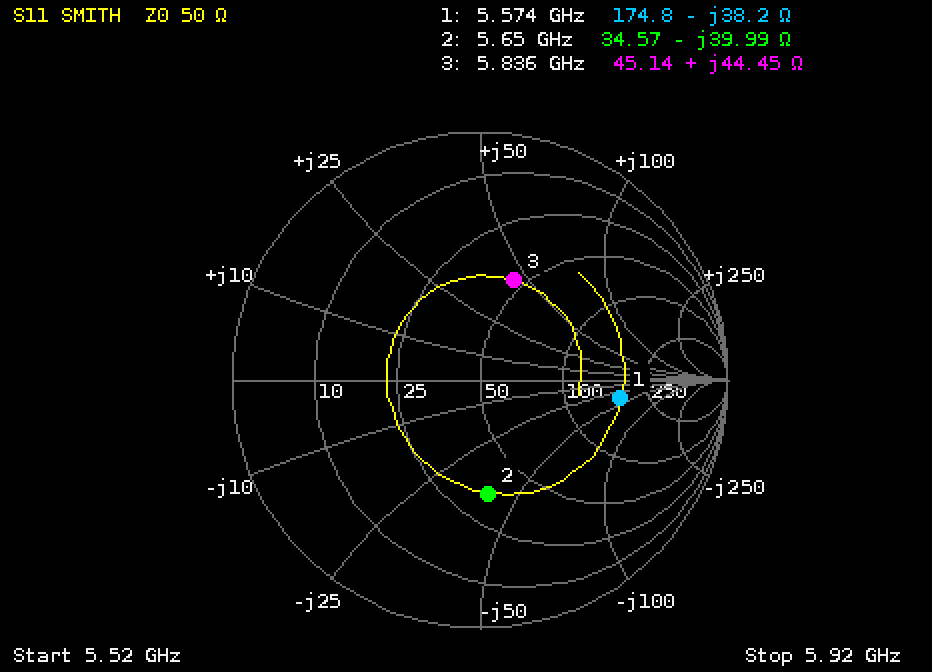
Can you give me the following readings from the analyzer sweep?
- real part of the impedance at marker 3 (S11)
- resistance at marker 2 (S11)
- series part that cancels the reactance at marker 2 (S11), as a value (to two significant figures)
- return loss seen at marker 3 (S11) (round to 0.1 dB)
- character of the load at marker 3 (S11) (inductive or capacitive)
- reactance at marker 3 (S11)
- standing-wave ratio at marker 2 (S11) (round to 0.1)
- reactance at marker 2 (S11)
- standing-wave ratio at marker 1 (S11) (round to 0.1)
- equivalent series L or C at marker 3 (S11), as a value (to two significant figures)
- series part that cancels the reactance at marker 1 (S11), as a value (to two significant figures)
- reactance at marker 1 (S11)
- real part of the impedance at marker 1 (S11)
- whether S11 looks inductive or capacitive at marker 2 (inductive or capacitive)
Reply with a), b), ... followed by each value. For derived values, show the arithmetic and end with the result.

a) 45.14 Ω
b) 34.57 Ω
c) L = 39.99 Ω/(2π × 5.65 GHz) ≈ 1.1 nH
d) 7.4 dB
e) inductive
f) +44.45 Ω
g) 2.7
h) -39.99 Ω
i) 3.7
j) L = 44.45 Ω/(2π × 5.836 GHz) ≈ 1.2 nH
k) L = 38.2 Ω/(2π × 5.574 GHz) ≈ 1.1 nH
l) -38.2 Ω
m) 174.8 Ω
n) capacitive
